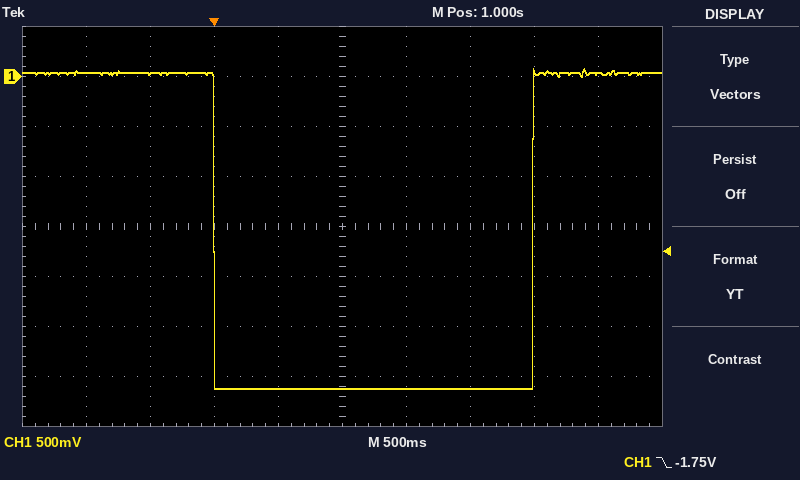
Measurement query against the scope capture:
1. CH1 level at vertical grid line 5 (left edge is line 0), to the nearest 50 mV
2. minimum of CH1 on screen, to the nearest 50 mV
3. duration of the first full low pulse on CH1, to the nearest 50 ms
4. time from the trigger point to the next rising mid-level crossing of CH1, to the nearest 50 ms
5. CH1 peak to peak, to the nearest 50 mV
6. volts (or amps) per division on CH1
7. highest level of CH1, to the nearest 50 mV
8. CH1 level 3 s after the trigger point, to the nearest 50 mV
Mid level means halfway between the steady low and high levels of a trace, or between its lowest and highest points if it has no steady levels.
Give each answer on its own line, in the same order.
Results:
-3.10 V
-3.10 V
2.50 s
2.50 s
3.20 V
500 mV
100 mV
50 mV
